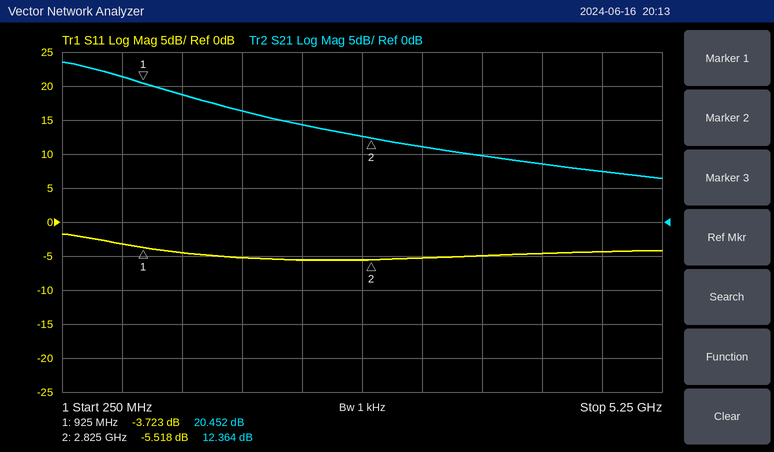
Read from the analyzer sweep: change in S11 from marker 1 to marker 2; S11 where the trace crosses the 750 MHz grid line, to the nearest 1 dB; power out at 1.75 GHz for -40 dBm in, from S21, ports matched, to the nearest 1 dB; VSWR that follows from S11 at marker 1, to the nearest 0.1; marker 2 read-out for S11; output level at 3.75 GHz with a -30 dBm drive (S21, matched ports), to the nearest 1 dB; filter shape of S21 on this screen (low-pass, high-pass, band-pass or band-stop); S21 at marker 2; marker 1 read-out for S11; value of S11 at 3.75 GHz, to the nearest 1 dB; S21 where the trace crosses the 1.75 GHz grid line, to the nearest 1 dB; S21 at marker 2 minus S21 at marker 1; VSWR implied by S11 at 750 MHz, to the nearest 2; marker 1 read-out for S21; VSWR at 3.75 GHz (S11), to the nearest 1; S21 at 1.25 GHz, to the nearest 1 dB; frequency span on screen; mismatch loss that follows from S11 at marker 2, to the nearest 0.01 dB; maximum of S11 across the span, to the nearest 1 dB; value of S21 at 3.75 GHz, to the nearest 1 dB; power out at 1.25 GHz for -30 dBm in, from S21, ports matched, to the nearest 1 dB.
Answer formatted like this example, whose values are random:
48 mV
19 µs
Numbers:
-1.795 dB
-3 dB
-24 dBm
4.7
-5.518 dB
-20 dBm
low-pass
12.364 dB
-3.723 dB
-5 dB
16 dB
-8.088 dB
6
20.452 dB
4
19 dB
5 GHz
1.43 dB
-2 dB
10 dB
-11 dBm
